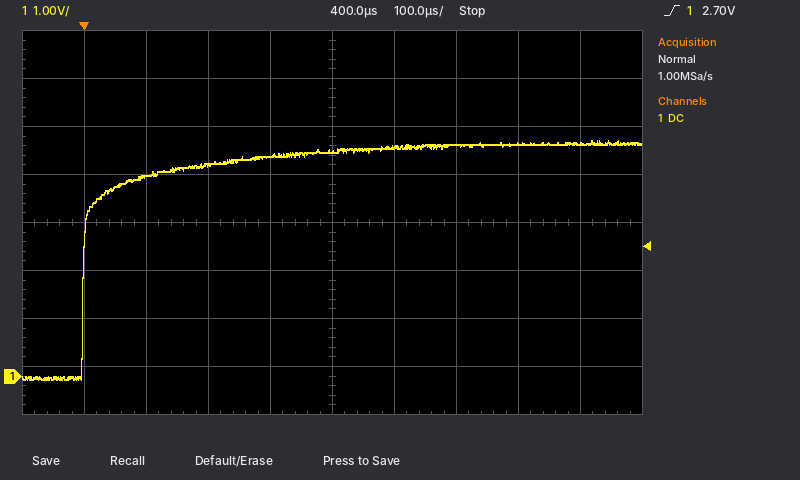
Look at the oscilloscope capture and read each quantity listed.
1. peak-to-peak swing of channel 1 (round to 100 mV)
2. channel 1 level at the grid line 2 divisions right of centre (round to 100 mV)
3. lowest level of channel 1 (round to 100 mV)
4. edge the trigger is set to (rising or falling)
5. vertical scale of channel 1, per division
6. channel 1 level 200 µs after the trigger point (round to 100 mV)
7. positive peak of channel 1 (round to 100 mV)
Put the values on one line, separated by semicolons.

5.0 V; 4.8 V; -100 mV; rising; 1 V; 4.4 V; 4.9 V
